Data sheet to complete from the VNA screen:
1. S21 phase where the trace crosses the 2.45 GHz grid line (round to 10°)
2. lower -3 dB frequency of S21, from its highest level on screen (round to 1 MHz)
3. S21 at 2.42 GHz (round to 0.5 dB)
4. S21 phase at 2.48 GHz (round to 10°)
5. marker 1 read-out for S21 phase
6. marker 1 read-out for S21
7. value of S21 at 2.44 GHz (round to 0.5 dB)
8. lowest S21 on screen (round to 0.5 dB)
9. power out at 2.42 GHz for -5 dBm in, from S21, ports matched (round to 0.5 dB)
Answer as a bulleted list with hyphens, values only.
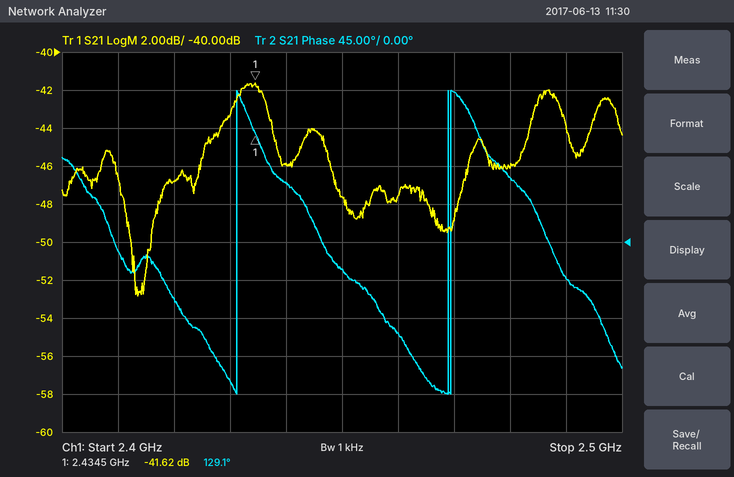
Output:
- -30°
- 2.427 GHz
- -47.0 dB
- 80°
- 129.1°
- -41.62 dB
- -46.0 dB
- -53.0 dB
- -52.0 dBm
